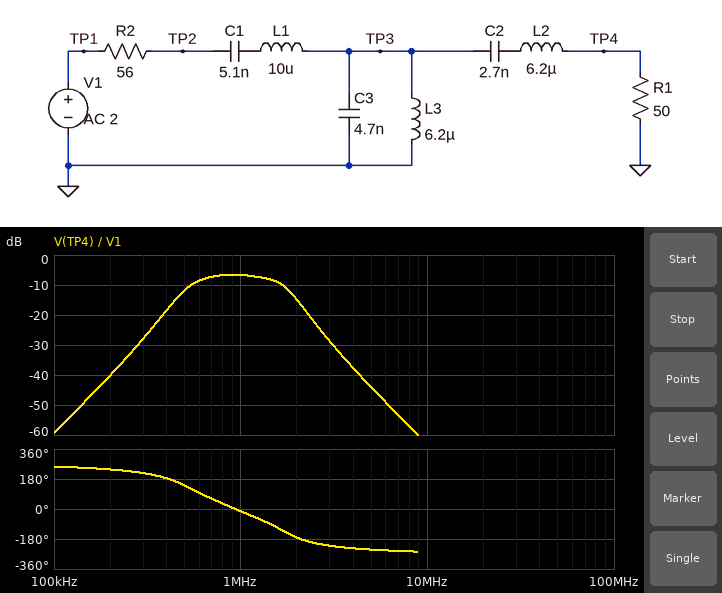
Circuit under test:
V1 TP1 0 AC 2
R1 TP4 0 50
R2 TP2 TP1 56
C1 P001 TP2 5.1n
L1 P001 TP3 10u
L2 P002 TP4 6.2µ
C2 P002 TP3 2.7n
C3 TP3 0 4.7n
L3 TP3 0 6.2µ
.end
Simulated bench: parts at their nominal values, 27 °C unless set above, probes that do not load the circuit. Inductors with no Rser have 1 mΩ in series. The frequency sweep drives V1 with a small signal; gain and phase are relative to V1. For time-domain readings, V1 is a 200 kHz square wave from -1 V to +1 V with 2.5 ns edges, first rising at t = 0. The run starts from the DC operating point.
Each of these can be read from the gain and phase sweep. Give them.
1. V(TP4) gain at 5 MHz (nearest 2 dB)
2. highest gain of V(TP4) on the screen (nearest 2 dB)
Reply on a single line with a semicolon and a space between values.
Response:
-44 dB; -6 dB
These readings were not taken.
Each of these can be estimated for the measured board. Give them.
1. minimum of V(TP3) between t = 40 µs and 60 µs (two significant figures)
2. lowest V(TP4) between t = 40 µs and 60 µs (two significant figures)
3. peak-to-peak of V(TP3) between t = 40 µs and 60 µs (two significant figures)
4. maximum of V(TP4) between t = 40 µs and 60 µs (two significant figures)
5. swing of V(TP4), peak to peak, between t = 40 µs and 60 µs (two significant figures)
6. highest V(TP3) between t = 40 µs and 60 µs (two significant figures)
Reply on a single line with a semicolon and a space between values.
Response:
-550 mV; -360 mV; 1.1 V; 360 mV; 720 mV; 550 mV
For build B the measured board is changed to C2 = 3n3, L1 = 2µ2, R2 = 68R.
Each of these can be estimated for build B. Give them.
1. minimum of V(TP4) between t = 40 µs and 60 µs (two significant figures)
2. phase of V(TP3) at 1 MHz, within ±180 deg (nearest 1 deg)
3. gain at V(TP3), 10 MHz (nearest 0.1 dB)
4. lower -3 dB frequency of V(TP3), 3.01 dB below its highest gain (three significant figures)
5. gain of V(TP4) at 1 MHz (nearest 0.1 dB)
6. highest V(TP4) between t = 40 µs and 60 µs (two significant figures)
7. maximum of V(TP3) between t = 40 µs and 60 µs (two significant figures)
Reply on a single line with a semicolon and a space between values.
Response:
-330 mV; -4 deg; -32.7 dB; 484 kHz; -7.9 dB; 330 mV; 560 mV
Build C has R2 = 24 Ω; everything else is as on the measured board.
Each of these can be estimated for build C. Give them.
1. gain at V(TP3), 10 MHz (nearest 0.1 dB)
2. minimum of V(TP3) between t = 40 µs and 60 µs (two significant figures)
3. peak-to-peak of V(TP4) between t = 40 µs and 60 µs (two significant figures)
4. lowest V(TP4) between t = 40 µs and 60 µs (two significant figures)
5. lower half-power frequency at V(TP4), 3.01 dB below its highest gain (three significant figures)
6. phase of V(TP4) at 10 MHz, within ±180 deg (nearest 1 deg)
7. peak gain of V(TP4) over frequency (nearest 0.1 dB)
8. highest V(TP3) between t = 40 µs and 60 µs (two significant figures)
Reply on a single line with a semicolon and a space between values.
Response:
-45.1 dB; -770 mV; 1.0 V; -510 mV; 481 kHz; 100 deg; -3.2 dB; 770 mV
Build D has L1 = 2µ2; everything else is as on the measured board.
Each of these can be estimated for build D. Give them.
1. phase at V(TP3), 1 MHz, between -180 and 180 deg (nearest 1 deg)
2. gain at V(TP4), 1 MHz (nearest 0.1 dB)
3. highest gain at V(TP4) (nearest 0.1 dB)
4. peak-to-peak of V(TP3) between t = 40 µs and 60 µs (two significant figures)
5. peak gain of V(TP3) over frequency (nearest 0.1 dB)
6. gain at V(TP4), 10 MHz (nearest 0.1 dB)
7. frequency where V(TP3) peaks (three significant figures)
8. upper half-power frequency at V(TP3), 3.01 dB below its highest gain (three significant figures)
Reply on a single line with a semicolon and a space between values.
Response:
-8 deg; -7.4 dB; -6.7 dB; 1.3 V; -2.4 dB; -50.1 dB; 622 kHz; 855 kHz
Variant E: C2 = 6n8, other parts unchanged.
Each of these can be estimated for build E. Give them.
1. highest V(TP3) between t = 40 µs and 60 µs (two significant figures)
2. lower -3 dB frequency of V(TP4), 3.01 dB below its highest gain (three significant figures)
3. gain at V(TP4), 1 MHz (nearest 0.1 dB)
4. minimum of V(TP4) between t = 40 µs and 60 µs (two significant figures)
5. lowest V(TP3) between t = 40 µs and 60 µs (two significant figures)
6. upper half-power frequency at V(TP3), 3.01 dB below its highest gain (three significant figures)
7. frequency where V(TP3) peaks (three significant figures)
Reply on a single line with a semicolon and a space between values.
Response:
490 mV; 448 kHz; -7.0 dB; -350 mV; -490 mV; 1.75 MHz; 1.39 MHz
